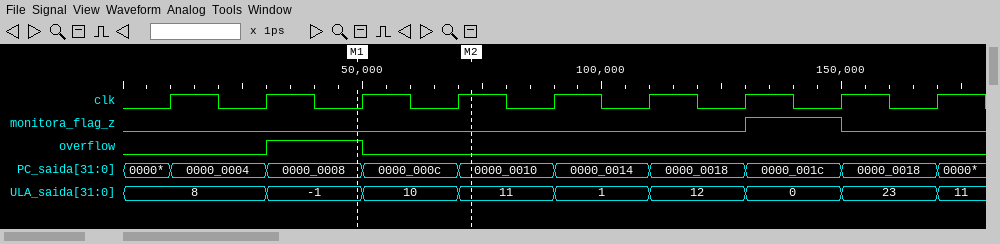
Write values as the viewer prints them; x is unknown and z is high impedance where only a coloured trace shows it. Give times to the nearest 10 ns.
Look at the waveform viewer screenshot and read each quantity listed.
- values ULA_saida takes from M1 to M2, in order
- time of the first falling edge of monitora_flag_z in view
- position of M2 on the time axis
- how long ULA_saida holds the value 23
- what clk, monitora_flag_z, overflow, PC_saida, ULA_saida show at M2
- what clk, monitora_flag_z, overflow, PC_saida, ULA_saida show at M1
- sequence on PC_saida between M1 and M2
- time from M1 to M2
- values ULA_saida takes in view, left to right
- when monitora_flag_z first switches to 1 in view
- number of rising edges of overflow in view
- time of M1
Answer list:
-1, 10, 11
150 ns
70 ns
20 ns
clk=1, monitora_flag_z=0, overflow=0, PC_saida=0000_0010, ULA_saida=11
clk=0, monitora_flag_z=0, overflow=1, PC_saida=0000_0008, ULA_saida=-1
0000_0008, 0000_000c, 0000_0010
20 ns
8, -1, 10, 11, 1, 12, 0, 23, 11
130 ns
1
50 ns
